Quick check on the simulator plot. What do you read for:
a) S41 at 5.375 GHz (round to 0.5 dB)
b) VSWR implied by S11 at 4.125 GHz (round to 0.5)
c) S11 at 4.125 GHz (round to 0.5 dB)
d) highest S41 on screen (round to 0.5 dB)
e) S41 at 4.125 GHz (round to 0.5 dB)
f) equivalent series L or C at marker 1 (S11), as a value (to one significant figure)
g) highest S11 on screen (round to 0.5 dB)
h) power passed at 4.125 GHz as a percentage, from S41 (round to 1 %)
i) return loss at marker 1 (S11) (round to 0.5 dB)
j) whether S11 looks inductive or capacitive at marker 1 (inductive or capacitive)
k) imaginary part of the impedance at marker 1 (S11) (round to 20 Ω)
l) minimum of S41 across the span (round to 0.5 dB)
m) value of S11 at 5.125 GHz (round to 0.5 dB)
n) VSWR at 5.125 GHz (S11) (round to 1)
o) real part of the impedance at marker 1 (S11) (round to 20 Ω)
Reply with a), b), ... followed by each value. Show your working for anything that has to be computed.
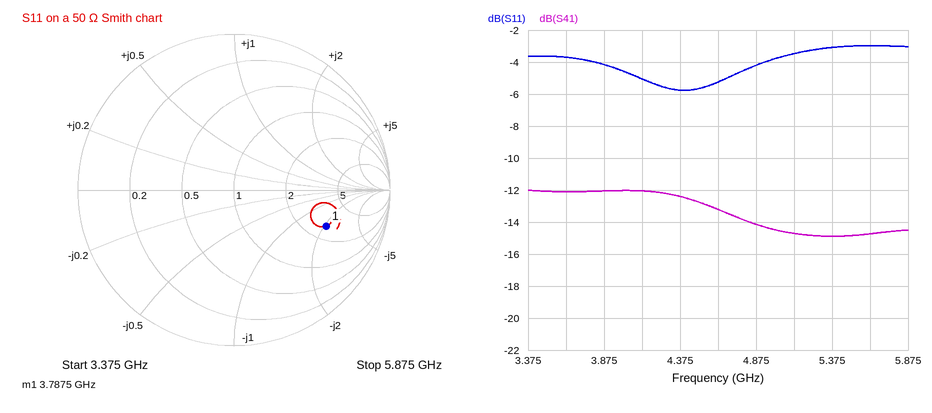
a) -15.0 dB
b) |Γ| = 10^(-5/20) = 0.5623; VSWR = (1 + 0.5623)/(1 − 0.5623) ≈ 3.57, so 3.5 to the nearest 0.5
c) -5.0 dB
d) -12.0 dB
e) -12.0 dB
f) C = 1/(2π × 3.7875 GHz × 100 Ω) ≈ 420 fF, so 400 fF to one significant figure
g) -3.0 dB
h) 10^(-12/10) ≈ 6 %
i) 4.0 dB
j) capacitive
k) -100 Ω
l) -15.0 dB
m) -3.5 dB
n) |Γ| = 10^(-3.5/20) = 0.6683; VSWR = (1 + 0.6683)/(1 − 0.6683) ≈ 5
o) 140 Ω
